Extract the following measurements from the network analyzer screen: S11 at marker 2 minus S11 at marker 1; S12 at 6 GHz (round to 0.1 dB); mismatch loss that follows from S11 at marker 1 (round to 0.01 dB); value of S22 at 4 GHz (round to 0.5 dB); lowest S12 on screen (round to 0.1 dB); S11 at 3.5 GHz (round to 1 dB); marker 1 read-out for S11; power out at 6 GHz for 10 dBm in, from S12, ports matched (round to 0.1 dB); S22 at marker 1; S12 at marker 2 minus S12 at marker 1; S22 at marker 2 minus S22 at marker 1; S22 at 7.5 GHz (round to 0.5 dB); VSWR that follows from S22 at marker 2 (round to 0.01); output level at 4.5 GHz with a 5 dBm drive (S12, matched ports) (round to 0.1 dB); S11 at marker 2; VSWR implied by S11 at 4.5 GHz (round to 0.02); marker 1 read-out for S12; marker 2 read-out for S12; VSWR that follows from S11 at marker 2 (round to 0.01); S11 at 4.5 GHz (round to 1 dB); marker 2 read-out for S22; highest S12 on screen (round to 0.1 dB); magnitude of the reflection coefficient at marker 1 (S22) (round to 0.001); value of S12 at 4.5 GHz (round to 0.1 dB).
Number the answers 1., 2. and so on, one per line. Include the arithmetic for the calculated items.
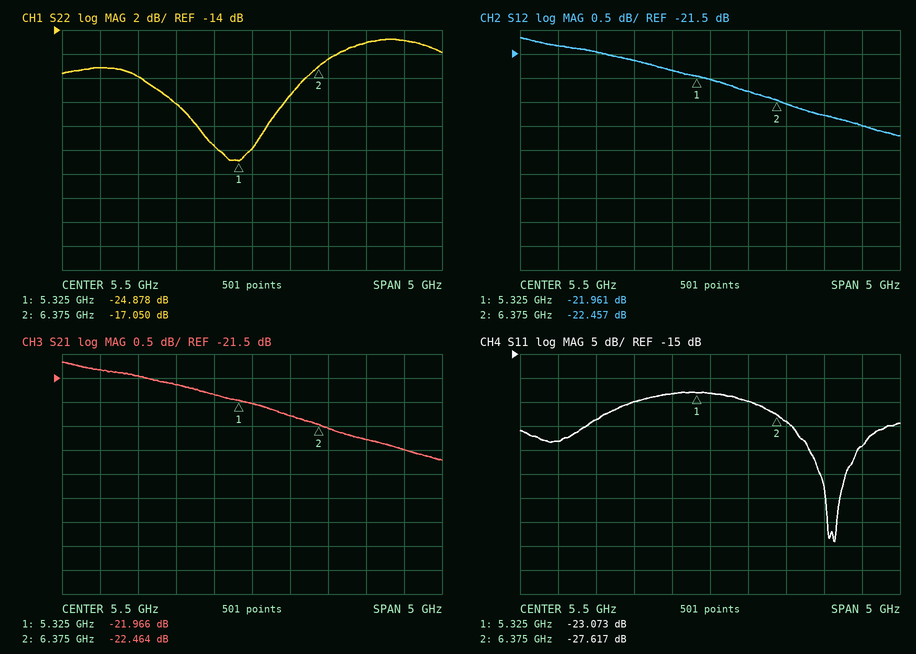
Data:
1. -27.617 − (-23.073) = -4.544 dB
2. -22.3 dB
3. −10 log10(1 − 10^(-23.073/10)) ≈ 0.02 dB
4. -18.0 dB
5. -23.2 dB
6. -33 dB
7. -23.073 dB
8. 10 dBm + (-22.3 dB) = -12.3 dBm
9. -24.878 dB
10. -22.457 − (-21.961) = -0.496 dB
11. -17.05 − (-24.878) = 7.828 dB
12. -15.0 dB
13. (1 + 0.1404)/(1 − 0.1404) ≈ 1.33
14. 5 dBm + (-21.6 dB) = -16.6 dBm
15. -27.617 dB
16. |Γ| = 10^(-25/20) = 0.0562; VSWR = (1 + 0.0562)/(1 − 0.0562) ≈ 1.12
17. -21.961 dB
18. -22.457 dB
19. (1 + 0.0416)/(1 − 0.0416) ≈ 1.09
20. -25 dB
21. -17.050 dB
22. -21.2 dB
23. 10^(-24.878/20) ≈ 0.057
24. -21.6 dB
